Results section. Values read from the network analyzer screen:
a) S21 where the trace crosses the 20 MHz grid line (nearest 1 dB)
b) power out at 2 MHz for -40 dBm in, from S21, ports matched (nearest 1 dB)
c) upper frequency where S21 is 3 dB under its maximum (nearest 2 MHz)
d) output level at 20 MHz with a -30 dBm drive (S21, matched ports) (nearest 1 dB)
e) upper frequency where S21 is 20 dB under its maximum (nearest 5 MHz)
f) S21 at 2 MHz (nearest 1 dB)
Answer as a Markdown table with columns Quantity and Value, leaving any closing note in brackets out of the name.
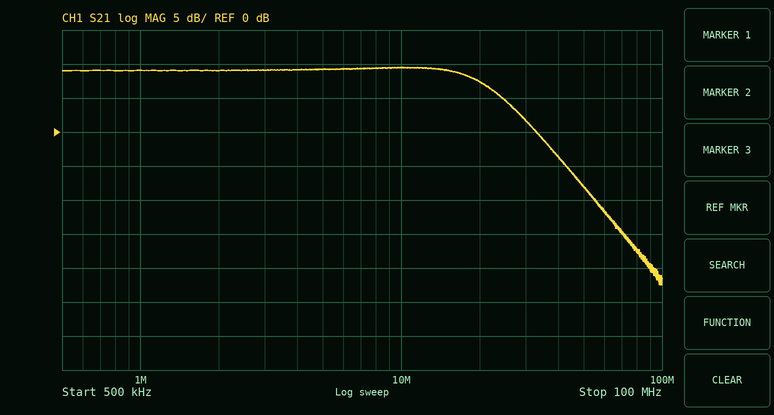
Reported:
| Quantity | Value |
|---|---|
| S21 where the trace crosses the 20 MHz grid line | 7 dB |
| power out at 2 MHz for -40 dBm in, from S21, ports matched | -31 dBm |
| upper frequency where S21 is 3 dB under its maximum | 22 MHz |
| output level at 20 MHz with a -30 dBm drive (S21, matched ports) | -23 dBm |
| upper frequency where S21 is 20 dB under its maximum | 55 MHz |
| S21 at 2 MHz | 9 dB |
